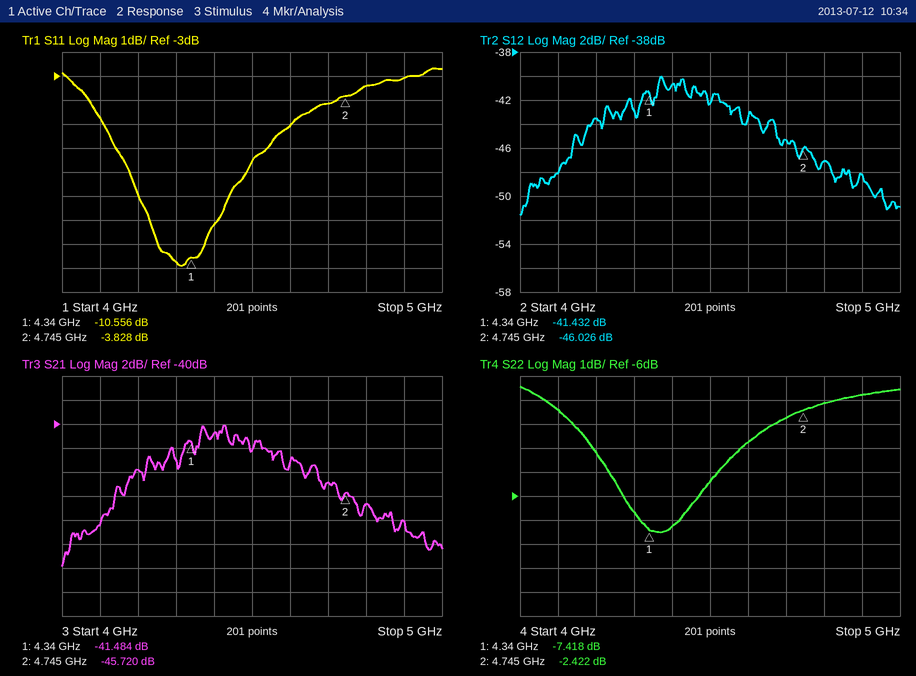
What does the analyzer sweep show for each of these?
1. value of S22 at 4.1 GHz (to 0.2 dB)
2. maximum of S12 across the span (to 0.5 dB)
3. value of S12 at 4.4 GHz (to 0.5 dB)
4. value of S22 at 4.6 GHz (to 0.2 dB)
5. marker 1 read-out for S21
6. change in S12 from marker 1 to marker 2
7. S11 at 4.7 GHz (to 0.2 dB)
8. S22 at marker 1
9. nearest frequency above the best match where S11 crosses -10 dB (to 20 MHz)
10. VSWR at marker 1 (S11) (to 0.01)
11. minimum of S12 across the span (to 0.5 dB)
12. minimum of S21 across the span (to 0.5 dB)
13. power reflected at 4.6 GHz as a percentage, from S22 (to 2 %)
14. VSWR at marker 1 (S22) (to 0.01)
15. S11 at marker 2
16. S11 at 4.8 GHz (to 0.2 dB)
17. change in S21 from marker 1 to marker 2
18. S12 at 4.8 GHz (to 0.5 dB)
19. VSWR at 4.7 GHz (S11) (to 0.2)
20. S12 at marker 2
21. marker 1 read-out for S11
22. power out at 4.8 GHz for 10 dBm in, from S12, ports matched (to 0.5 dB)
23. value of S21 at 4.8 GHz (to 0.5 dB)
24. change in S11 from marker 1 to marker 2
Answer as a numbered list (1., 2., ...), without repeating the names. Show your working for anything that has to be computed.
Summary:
1. -2.4 dB
2. -40.0 dB
3. -40.5 dB
4. -3.8 dB
5. -41.484 dB
6. -46.026 − (-41.432) = -4.594 dB
7. -4.2 dB
8. -7.418 dB
9. 4.38 GHz
10. (1 + 0.2966)/(1 − 0.2966) ≈ 1.84
11. -51.5 dB
12. -52.0 dB
13. 10^(-3.8/10) ≈ 42 %
14. (1 + 0.4257)/(1 − 0.4257) ≈ 2.48
15. -3.828 dB
16. -3.4 dB
17. -45.72 − (-41.484) = -4.236 dB
18. -47.0 dB
19. |Γ| = 10^(-4.2/20) = 0.6166; VSWR = (1 + 0.6166)/(1 − 0.6166) ≈ 4.2
20. -46.026 dB
21. -10.556 dB
22. 10 dBm + (-47.0 dB) = -37.0 dBm
23. -46.5 dB
24. -3.828 − (-10.556) = 6.728 dB
